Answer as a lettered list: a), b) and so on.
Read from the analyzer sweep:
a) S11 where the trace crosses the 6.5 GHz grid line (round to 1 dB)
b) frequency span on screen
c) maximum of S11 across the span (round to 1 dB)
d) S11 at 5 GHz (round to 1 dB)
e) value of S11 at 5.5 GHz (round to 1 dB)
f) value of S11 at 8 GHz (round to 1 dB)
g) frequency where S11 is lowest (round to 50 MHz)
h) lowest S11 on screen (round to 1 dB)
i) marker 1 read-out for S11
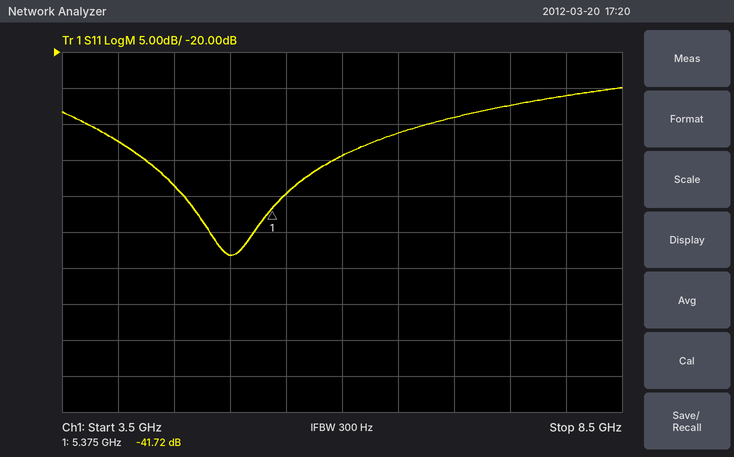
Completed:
a) -31 dB
b) 5 GHz
c) -25 dB
d) -48 dB
e) -40 dB
f) -26 dB
g) 5.00 GHz
h) -48 dB
i) -41.72 dB
